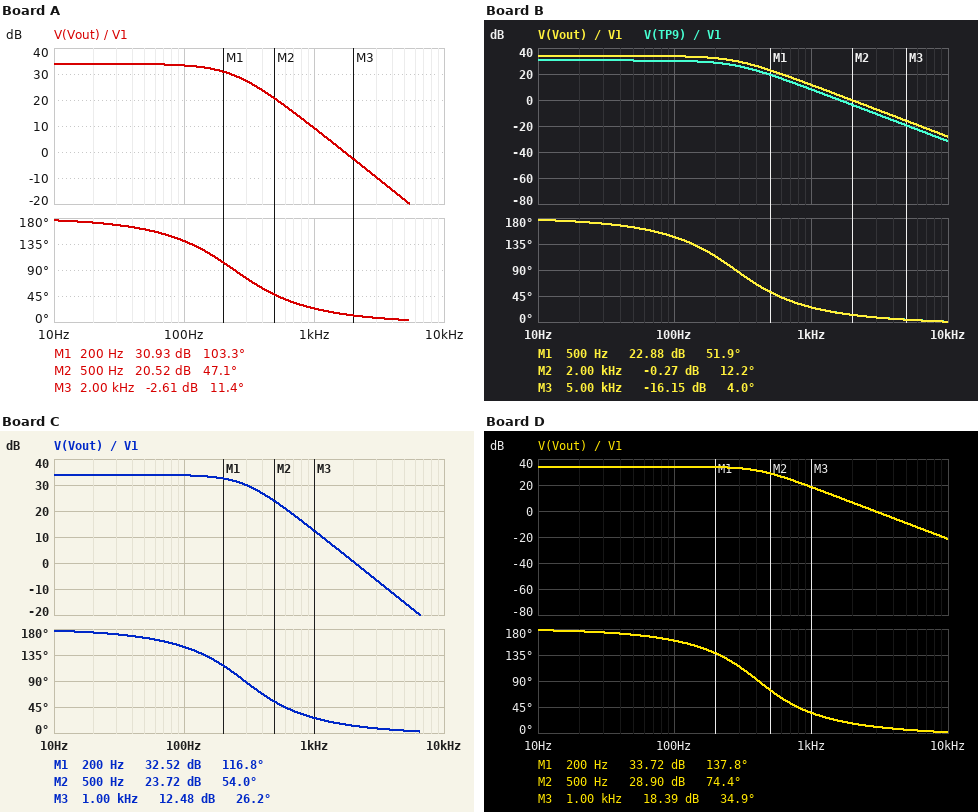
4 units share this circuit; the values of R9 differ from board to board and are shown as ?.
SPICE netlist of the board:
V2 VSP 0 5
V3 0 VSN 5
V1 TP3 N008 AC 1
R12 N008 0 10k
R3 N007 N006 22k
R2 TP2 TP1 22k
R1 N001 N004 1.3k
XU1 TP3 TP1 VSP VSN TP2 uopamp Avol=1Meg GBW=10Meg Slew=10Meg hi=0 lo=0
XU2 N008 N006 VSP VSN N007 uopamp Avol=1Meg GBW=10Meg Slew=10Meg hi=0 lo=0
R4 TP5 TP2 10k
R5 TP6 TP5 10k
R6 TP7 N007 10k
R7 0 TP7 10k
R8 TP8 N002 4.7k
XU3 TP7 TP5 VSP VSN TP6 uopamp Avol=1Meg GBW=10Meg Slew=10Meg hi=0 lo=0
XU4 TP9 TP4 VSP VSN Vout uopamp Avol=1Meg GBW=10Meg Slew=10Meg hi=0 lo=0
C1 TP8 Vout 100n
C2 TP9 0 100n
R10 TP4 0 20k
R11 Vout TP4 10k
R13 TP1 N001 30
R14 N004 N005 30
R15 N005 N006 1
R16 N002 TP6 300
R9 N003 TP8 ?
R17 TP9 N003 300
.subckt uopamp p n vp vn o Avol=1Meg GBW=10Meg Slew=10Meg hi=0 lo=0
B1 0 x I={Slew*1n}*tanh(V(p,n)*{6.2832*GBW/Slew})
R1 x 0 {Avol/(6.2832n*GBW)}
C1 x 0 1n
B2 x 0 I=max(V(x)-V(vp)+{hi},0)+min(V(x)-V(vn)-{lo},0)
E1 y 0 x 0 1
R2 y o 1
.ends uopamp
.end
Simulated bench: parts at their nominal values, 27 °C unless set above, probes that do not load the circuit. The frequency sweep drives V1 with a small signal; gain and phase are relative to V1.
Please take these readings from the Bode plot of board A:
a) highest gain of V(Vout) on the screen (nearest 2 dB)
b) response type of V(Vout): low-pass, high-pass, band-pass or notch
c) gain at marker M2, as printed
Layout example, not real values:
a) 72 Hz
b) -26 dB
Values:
a) 34 dB
b) low-pass
c) 20.52 dB
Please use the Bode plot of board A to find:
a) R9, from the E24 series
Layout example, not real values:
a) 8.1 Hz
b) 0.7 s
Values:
a) 8.2 kΩ
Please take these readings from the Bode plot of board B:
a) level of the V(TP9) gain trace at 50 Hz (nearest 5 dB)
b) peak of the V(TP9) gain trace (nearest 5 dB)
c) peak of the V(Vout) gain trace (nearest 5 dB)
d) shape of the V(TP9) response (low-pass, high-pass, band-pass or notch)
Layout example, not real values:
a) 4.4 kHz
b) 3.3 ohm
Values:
a) 30 dB
b) 30 dB
c) 35 dB
d) low-pass
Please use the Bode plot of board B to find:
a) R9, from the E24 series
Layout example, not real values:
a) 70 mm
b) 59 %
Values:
a) 6.2 kΩ
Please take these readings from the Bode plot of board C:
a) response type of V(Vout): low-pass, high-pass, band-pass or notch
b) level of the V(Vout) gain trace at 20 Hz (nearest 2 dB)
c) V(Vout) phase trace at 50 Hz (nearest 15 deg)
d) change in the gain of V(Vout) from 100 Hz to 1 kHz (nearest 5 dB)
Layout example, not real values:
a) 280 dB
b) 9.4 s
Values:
a) low-pass
b) 34 dB
c) 165 deg
d) -20 dB
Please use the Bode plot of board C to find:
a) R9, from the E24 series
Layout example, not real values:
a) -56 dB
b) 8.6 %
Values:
a) 5.6 kΩ
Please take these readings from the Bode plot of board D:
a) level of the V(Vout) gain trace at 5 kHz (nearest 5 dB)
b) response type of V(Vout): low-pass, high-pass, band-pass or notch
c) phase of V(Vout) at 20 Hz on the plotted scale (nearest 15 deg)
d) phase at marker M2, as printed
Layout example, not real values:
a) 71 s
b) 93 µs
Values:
a) -10 dB
b) low-pass
c) 180 deg
d) 74.4 deg
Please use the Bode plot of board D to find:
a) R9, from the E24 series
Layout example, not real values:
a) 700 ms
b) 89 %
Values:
a) 2.7 kΩ
